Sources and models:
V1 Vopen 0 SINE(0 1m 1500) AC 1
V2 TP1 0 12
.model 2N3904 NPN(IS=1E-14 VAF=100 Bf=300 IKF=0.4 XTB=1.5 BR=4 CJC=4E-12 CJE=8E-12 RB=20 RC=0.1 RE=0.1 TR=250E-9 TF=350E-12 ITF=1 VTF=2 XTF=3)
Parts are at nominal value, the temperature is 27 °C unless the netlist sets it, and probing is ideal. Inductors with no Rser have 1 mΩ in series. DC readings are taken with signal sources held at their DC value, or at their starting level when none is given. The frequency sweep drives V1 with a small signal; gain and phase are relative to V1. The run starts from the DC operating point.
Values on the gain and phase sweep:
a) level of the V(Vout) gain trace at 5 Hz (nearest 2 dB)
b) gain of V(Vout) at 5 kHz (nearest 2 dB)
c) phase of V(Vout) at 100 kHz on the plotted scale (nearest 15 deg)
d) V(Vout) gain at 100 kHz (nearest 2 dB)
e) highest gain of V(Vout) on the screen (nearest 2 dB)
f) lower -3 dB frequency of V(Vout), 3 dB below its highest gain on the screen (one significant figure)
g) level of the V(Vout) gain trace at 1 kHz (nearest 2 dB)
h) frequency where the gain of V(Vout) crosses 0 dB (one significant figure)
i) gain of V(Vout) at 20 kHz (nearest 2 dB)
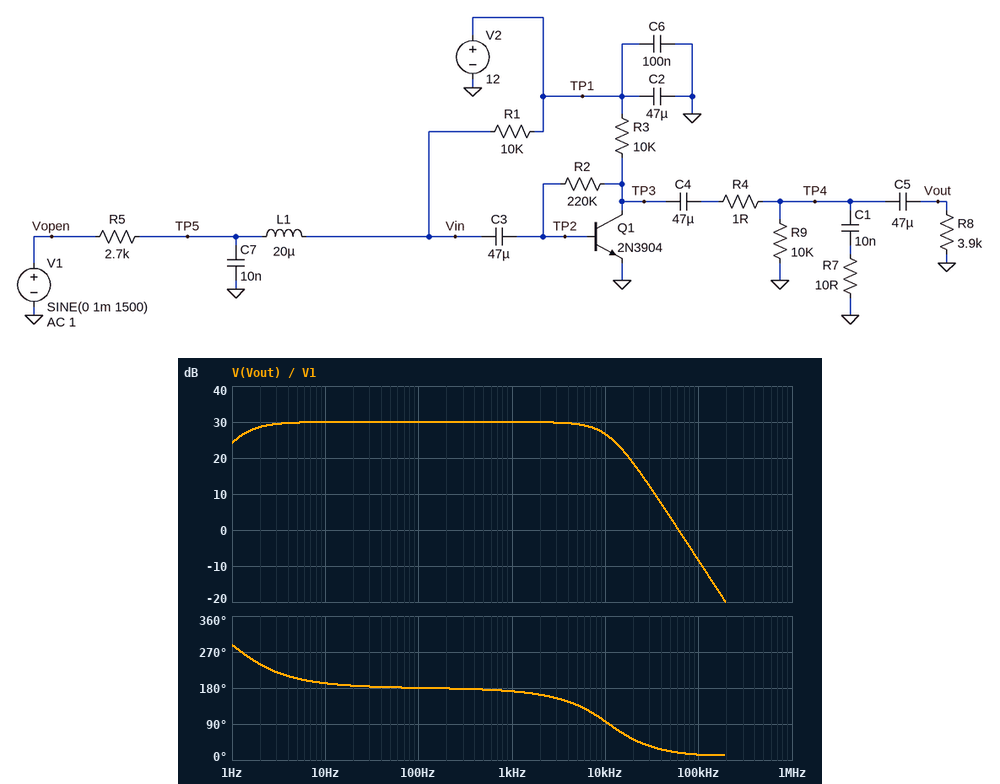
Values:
30 dB
30 dB
15 deg
-8 dB
30 dB
1 Hz
30 dB
60 kHz
18 dB
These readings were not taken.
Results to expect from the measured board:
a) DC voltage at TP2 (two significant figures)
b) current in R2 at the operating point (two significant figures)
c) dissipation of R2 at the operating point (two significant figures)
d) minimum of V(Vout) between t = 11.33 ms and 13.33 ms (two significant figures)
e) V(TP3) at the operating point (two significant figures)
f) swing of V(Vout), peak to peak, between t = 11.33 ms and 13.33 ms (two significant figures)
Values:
660 mV
3.5 µA
2.7 µW
-32 mV
1.4 V
63 mV
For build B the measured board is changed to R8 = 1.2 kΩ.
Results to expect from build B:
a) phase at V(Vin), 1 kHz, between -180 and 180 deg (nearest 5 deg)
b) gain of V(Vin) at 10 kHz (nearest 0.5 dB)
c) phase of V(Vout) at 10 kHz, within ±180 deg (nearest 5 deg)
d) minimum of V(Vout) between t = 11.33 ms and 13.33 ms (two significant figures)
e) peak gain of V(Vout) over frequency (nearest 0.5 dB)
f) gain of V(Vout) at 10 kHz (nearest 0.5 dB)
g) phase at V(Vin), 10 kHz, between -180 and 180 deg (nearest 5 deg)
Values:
-5 deg
-8.0 dB
110 deg
-18 mV
25.0 dB
22.5 dB
-35 deg
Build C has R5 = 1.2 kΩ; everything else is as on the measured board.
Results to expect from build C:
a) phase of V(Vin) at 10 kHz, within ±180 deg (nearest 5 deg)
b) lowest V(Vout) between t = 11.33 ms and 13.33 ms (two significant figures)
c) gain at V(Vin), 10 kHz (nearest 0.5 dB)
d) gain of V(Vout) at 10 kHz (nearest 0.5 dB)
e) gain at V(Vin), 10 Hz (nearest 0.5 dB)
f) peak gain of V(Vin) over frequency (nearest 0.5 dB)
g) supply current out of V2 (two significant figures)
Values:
-20 deg
-49 mV
-4.0 dB
30.5 dB
-5.0 dB
-1.0 dB
2.1 mA
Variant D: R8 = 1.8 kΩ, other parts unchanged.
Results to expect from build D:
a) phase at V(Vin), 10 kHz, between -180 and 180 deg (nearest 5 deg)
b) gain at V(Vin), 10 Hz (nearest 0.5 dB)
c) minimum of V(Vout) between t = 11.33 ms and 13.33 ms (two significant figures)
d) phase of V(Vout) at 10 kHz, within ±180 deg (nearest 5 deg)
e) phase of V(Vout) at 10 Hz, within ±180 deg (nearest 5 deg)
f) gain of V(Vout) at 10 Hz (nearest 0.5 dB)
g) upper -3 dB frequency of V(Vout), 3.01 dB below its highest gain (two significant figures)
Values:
-35 deg
-7.5 dB
-23 mV
105 deg
-165 deg
27.0 dB
10 kHz
